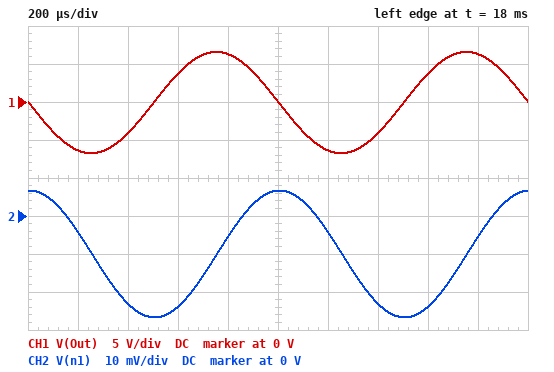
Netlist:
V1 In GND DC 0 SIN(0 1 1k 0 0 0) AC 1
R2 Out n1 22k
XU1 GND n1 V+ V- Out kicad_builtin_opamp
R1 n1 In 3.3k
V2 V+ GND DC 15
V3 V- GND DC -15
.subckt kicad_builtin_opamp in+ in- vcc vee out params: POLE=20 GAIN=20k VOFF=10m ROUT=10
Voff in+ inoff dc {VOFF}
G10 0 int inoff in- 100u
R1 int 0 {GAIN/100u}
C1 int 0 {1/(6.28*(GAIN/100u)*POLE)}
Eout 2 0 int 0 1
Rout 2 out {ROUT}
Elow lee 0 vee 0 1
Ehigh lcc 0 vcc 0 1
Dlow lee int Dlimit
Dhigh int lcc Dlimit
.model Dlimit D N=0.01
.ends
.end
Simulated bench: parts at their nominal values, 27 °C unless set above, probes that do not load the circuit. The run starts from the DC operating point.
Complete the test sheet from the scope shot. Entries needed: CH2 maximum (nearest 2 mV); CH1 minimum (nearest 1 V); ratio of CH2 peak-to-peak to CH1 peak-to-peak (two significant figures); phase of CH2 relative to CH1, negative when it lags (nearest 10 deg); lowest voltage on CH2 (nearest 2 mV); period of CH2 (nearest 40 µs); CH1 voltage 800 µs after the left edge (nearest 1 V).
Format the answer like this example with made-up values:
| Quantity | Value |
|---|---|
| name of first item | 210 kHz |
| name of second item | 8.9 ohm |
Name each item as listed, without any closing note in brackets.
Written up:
| Quantity | Value |
|---|---|
| CH2 maximum | 6 mV |
| CH1 minimum | -7 V |
| ratio of CH2 peak-to-peak to CH1 peak-to-peak | 0.0025 |
| phase of CH2 relative to CH1, negative when it lags | -90 deg |
| lowest voltage on CH2 | -26 mV |
| period of CH2 | 1.00 ms |
| CH1 voltage 800 µs after the left edge | 6 V |
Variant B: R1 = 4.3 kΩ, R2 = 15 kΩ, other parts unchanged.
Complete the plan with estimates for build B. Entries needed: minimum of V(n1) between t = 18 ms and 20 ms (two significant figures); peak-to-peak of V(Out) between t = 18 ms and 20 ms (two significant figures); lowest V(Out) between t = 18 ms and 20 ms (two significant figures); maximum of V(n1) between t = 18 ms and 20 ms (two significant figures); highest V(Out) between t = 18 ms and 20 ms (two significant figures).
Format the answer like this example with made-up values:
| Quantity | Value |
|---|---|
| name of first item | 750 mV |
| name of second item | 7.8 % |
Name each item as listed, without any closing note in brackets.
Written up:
| Quantity | Value |
|---|---|
| minimum of V(n1) between t = 18 ms and 20 ms | -19 mV |
| peak-to-peak of V(Out) between t = 18 ms and 20 ms | 7.0 V |
| lowest V(Out) between t = 18 ms and 20 ms | -3.5 V |
| maximum of V(n1) between t = 18 ms and 20 ms | -1.3 mV |
| highest V(Out) between t = 18 ms and 20 ms | 3.4 V |
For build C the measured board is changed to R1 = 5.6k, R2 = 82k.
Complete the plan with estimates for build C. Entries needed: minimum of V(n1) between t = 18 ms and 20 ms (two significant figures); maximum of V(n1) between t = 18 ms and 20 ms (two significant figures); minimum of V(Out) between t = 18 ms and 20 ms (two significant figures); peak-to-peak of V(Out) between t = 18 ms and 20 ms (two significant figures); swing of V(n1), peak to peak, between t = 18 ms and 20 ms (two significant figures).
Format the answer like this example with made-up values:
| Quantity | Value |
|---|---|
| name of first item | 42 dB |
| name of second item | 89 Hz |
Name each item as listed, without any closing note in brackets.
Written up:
| Quantity | Value |
|---|---|
| minimum of V(n1) between t = 18 ms and 20 ms | -47 mV |
| maximum of V(n1) between t = 18 ms and 20 ms | 27 mV |
| minimum of V(Out) between t = 18 ms and 20 ms | -15 V |
| peak-to-peak of V(Out) between t = 18 ms and 20 ms | 29 V |
| swing of V(n1), peak to peak, between t = 18 ms and 20 ms | 73 mV |
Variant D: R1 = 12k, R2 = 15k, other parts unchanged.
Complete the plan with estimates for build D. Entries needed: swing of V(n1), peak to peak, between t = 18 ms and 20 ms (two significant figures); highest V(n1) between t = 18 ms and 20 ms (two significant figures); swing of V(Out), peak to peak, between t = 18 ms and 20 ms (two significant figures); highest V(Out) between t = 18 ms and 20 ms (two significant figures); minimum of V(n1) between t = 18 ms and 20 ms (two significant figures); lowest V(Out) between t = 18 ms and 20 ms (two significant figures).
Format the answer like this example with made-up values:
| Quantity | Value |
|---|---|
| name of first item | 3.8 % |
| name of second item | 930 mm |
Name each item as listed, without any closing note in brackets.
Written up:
| Quantity | Value |
|---|---|
| swing of V(n1), peak to peak, between t = 18 ms and 20 ms | 6.3 mV |
| highest V(n1) between t = 18 ms and 20 ms | -6.9 mV |
| swing of V(Out), peak to peak, between t = 18 ms and 20 ms | 2.5 V |
| highest V(Out) between t = 18 ms and 20 ms | 1.2 V |
| minimum of V(n1) between t = 18 ms and 20 ms | -13 mV |
| lowest V(Out) between t = 18 ms and 20 ms | -1.3 V |
